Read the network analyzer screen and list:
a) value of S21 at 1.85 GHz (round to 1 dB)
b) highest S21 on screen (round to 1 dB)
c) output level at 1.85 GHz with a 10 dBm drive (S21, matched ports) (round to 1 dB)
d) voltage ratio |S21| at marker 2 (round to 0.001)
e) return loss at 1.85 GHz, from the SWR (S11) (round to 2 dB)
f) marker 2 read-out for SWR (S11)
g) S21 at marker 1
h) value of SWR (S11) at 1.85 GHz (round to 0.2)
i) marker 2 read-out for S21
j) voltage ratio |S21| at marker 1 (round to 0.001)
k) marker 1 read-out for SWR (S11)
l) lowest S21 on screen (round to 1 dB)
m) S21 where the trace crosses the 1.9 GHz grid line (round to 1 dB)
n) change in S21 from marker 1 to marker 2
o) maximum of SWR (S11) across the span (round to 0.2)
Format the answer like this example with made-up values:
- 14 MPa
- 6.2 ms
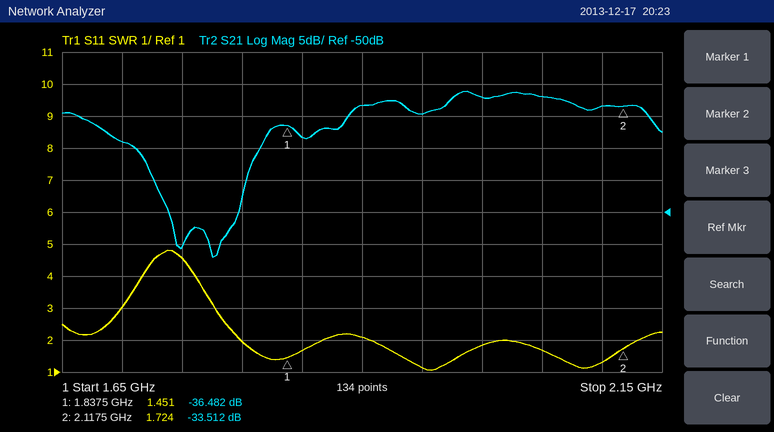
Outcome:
- -38 dB
- -31 dB
- -28 dBm
- 0.021
- 12 dB
- 1.724
- -36.482 dB
- 1.6
- -33.512 dB
- 0.015
- 1.451
- -57 dB
- -33 dB
- 2.970 dB
- 4.8
